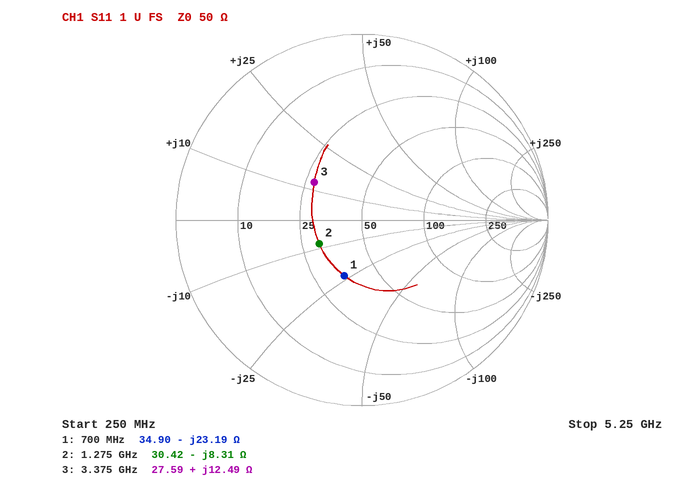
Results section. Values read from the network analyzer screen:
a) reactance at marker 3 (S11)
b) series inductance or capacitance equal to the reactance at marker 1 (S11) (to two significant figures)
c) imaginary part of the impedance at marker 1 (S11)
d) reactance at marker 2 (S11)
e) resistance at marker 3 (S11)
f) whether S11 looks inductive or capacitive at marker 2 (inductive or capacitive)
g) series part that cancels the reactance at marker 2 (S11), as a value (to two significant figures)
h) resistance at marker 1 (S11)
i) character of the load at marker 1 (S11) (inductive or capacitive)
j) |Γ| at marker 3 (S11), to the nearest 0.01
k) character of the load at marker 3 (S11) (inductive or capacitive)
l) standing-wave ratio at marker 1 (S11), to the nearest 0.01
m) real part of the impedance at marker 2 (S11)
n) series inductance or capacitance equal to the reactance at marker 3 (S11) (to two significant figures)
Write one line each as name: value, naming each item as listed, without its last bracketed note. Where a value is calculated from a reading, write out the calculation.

reactance at marker 3: +12.49 Ω
series inductance or capacitance equal to the reactance at marker 1 (S11): C = 1/(2π × 700 MHz × 23.19 Ω) ≈ 9.8 pF
imaginary part of the impedance at marker 1: -23.19 Ω
reactance at marker 2: -8.31 Ω
resistance at marker 3: 27.59 Ω
whether S11 looks inductive or capacitive at marker 2: capacitive
series part that cancels the reactance at marker 2 (S11), as a value: L = 8.31 Ω/(2π × 1.275 GHz) ≈ 1.0 nH
resistance at marker 1: 34.90 Ω
character of the load at marker 1 (S11): capacitive
|Γ| at marker 3 (S11), to the nearest 0.01: 0.33
character of the load at marker 3 (S11): inductive
standing-wave ratio at marker 1 (S11), to the nearest 0.01: 1.92
real part of the impedance at marker 2: 30.42 Ω
series inductance or capacitance equal to the reactance at marker 3 (S11): L = 12.49 Ω/(2π × 3.375 GHz) ≈ 589 pH, so 590 pH to two significant figures
